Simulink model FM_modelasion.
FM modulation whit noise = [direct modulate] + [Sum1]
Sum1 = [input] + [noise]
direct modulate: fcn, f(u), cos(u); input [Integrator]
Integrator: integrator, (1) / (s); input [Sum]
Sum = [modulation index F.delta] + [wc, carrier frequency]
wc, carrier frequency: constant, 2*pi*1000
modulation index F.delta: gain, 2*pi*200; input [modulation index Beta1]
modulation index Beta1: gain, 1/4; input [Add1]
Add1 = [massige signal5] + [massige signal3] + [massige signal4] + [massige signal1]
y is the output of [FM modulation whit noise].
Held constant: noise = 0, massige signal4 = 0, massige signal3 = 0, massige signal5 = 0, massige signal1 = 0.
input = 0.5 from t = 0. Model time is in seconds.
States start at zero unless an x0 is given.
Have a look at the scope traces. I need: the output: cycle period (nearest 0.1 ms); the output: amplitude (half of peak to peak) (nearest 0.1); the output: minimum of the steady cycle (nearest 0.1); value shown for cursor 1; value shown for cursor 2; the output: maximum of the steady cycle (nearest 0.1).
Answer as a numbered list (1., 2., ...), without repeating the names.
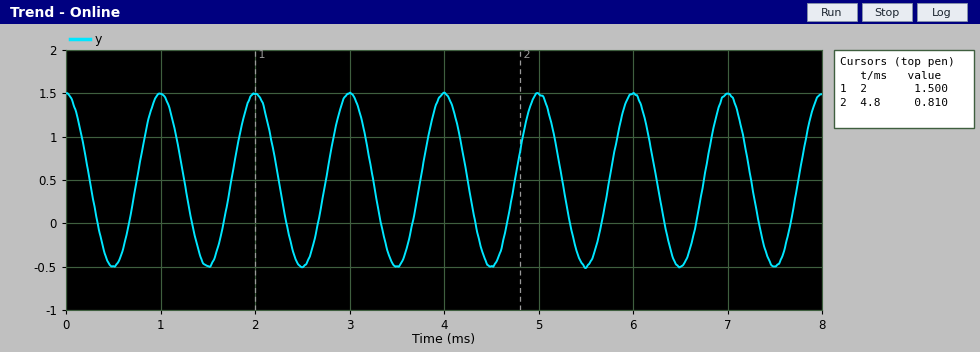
1. 1.0 ms
2. 1.0
3. -0.5
4. 1.500
5. 0.810
6. 1.5
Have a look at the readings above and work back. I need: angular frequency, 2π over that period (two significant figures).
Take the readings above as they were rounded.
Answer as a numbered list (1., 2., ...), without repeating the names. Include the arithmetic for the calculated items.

1. 2π / 1 = 6.3 rad/ms
